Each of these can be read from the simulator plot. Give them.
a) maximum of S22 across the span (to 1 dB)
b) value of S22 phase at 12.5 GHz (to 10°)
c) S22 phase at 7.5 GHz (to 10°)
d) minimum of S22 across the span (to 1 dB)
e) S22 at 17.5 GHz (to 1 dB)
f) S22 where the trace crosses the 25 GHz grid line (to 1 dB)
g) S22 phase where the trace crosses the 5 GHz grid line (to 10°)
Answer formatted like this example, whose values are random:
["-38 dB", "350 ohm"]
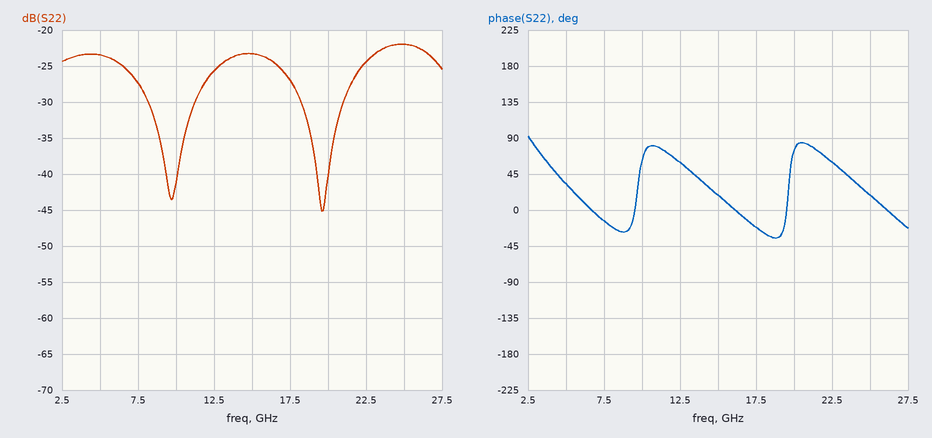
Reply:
["-22 dB", "60°", "-10°", "-45 dB", "-27 dB", "-22 dB", "30°"]
